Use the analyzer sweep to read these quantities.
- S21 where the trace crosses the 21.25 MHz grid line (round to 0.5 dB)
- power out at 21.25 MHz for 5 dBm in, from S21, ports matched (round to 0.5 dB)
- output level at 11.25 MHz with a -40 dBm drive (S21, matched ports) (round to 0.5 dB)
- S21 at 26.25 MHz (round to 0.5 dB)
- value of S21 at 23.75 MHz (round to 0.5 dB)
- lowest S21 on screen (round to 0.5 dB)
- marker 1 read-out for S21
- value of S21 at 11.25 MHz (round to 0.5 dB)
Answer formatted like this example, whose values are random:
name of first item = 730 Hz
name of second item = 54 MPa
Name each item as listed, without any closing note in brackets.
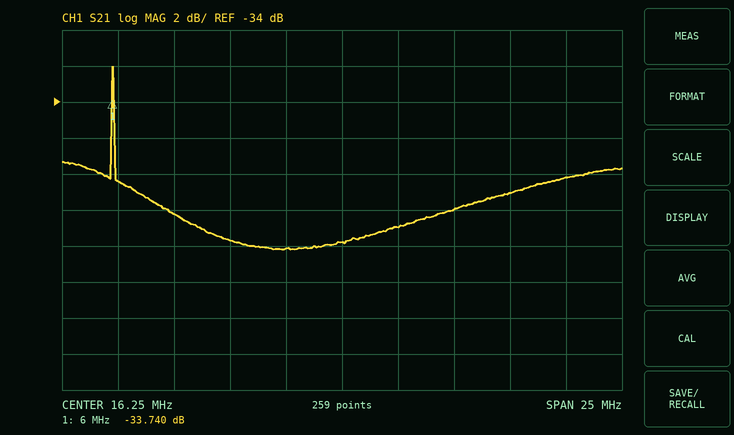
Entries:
S21 where the trace crosses the 21.25 MHz grid line = -40.0 dB
power out at 21.25 MHz for 5 dBm in, from S21, ports matched = -35.0 dBm
output level at 11.25 MHz with a -40 dBm drive (S21, matched ports) = -81.5 dBm
S21 at 26.25 MHz = -38.0 dB
value of S21 at 23.75 MHz = -39.0 dB
lowest S21 on screen = -42.0 dB
marker 1 read-out for S21 = -33.740 dB
value of S21 at 11.25 MHz = -41.5 dB
